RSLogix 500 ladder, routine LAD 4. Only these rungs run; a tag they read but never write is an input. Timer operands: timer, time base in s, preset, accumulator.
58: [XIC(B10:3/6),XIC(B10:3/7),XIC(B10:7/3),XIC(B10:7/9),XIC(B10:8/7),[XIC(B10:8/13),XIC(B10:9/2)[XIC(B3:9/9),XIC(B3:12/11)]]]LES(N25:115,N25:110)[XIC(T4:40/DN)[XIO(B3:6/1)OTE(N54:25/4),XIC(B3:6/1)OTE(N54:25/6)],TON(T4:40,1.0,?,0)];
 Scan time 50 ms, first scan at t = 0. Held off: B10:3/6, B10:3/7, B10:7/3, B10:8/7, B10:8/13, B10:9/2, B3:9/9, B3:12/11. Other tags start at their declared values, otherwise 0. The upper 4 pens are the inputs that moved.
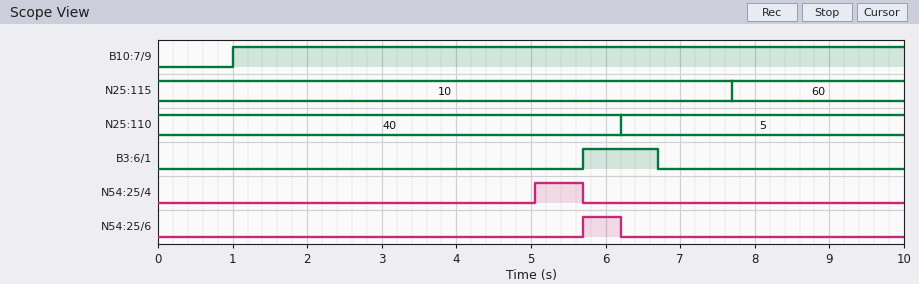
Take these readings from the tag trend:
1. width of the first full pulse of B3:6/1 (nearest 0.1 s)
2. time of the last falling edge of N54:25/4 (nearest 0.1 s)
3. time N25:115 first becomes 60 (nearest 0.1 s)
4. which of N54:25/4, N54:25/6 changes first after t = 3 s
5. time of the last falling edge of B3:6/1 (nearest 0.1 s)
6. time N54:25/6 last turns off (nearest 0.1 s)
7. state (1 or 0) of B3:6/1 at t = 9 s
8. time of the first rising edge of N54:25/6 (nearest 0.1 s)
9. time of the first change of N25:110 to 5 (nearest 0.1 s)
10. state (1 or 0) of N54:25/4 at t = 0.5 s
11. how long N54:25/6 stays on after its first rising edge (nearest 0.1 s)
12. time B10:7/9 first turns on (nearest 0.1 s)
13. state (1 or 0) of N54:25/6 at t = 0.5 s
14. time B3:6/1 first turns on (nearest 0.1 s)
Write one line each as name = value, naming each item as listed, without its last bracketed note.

width of the first full pulse of B3:6/1 = 1.0 s
time of the last falling edge of N54:25/4 = 5.7 s
time N25:115 first becomes 60 = 7.7 s
which of N54:25/4, N54:25/6 changes first after t = 3 s = N54:25/4
time of the last falling edge of B3:6/1 = 6.7 s
time N54:25/6 last turns off = 6.2 s
state (1 or 0) of B3:6/1 at t = 9 s = 0
time of the first rising edge of N54:25/6 = 5.7 s
time of the first change of N25:110 to 5 = 6.2 s
state (1 or 0) of N54:25/4 at t = 0.5 s = 0
how long N54:25/6 stays on after its first rising edge = 0.5 s
time B10:7/9 first turns on = 1.0 s
state (1 or 0) of N54:25/6 at t = 0.5 s = 0
time B3:6/1 first turns on = 5.7 s
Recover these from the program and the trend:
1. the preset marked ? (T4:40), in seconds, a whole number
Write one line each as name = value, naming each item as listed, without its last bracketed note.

the preset marked ? (T4:40), in seconds, a whole number = 4 s
